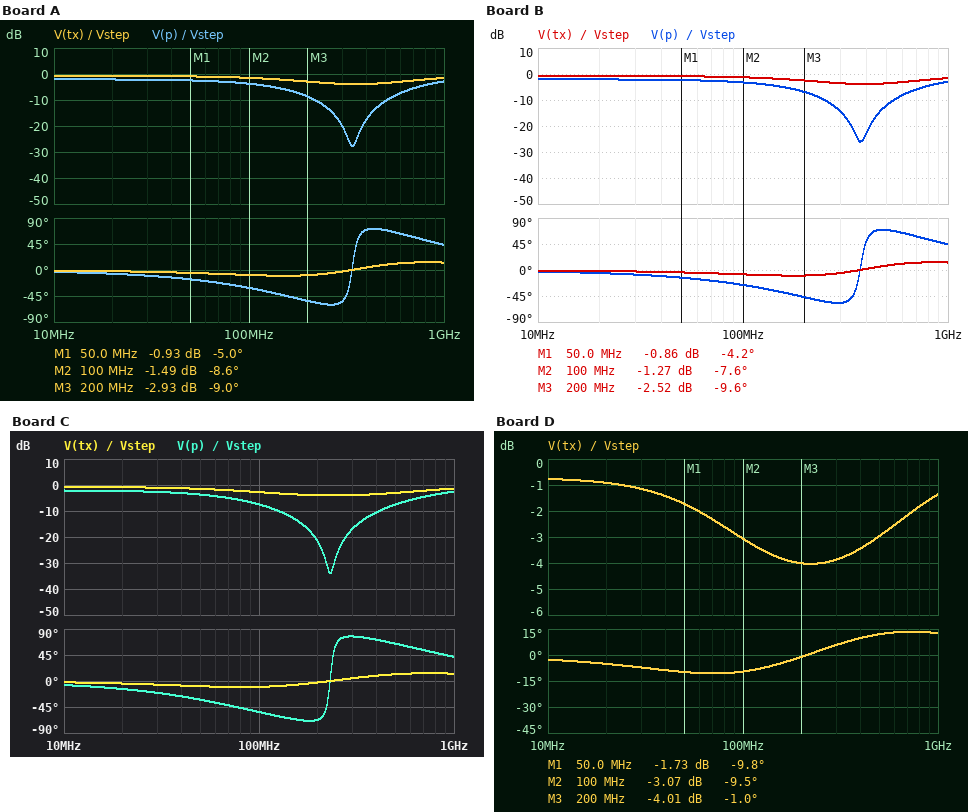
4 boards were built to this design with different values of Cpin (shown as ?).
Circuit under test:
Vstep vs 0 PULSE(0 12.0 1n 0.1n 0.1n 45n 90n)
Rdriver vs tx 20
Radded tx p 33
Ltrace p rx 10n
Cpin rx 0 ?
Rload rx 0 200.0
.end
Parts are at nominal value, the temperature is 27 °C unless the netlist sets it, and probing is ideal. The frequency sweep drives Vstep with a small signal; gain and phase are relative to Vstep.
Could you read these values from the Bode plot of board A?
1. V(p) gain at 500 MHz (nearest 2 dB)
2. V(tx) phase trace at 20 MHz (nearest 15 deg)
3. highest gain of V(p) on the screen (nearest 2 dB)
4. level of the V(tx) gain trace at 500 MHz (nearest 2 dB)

-10 dB
0 deg
-2 dB
-4 dB
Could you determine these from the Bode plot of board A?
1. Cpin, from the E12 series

22 pF
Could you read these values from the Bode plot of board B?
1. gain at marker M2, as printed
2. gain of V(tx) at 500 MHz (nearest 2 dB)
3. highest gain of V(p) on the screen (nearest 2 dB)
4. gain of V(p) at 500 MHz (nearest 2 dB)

-1.27 dB
-4 dB
-2 dB
-12 dB
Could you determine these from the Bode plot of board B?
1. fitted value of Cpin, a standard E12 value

18 pF
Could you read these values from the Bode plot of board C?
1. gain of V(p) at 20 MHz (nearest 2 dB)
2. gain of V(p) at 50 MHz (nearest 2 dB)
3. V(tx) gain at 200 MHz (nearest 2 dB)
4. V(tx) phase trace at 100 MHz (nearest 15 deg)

-2 dB
-4 dB
-4 dB
-15 deg
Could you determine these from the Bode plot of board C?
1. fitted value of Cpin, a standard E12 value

47 pF
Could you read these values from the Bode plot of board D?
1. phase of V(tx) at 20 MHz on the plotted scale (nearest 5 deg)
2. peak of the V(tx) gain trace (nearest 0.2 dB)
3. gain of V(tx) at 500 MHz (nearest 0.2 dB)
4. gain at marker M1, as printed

-5 deg
-0.8 dB
-3.0 dB
-1.73 dB
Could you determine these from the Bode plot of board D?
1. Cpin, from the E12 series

56 pF
